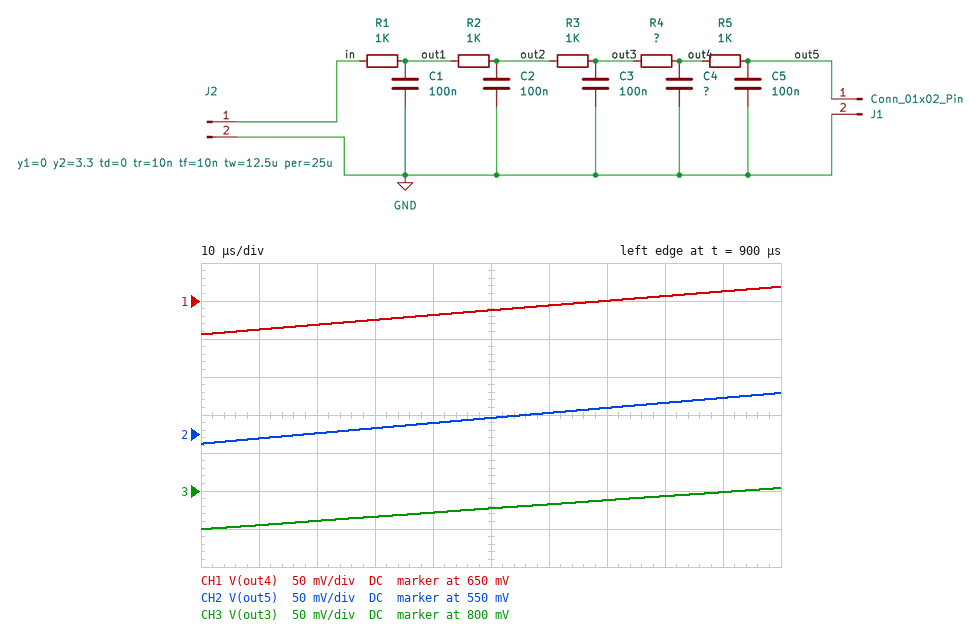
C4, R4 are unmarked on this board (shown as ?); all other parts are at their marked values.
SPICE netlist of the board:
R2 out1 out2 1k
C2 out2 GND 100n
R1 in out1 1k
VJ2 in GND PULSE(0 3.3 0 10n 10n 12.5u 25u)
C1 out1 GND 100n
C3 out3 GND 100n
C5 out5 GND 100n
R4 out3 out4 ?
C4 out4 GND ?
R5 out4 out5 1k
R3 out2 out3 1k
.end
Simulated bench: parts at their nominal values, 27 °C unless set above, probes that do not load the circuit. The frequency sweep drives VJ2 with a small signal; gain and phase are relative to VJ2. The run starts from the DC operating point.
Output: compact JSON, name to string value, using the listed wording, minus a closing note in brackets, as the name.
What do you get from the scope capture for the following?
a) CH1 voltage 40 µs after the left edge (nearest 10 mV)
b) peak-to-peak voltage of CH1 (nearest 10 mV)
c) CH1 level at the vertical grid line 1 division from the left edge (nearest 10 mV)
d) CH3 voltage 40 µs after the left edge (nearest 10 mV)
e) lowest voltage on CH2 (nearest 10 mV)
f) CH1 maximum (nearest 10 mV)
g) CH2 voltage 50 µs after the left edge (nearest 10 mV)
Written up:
{"CH1 voltage 40 µs after the left edge": "630 mV", "peak-to-peak voltage of CH1": "60 mV", "CH1 level at the vertical grid line 1 division from the left edge": "610 mV", "CH3 voltage 40 µs after the left edge": "770 mV", "lowest voltage on CH2": "540 mV", "CH1 maximum": "670 mV", "CH2 voltage 50 µs after the left edge": "570 mV"}
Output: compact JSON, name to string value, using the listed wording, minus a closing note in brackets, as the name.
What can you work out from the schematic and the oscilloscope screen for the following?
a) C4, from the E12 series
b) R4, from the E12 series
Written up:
{"C4, from the E12 series": "220 nF", "R4, from the E12 series": "680 Ω"}
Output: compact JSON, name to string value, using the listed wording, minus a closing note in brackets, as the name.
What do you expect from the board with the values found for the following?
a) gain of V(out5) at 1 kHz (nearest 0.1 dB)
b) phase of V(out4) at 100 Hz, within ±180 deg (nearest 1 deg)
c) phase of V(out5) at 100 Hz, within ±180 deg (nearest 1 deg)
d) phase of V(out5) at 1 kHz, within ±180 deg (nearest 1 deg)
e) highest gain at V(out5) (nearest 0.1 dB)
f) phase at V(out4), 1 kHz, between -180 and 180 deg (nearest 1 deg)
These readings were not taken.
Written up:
{"gain of V(out5) at 1 kHz": "-23.5 dB", "phase of V(out4) at 100 Hz, within ±180 deg": "-51 deg", "phase of V(out5) at 100 Hz, within ±180 deg": "-55 deg", "phase of V(out5) at 1 kHz, within ±180 deg": "-170 deg", "highest gain at V(out5)": "0 dB", "phase at V(out4), 1 kHz, between -180 and 180 deg": "-138 deg"}
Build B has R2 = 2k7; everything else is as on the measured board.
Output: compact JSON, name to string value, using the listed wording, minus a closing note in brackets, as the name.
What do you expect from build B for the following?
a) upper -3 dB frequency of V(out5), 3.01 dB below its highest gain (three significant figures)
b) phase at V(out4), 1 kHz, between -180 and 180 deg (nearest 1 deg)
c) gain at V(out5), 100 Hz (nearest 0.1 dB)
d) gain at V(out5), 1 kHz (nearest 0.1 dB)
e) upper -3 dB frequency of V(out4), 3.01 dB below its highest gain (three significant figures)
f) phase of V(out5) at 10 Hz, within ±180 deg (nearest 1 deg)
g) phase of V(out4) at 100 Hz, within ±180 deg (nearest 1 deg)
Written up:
{"upper -3 dB frequency of V(out5), 3.01 dB below its highest gain": "64.2 Hz", "phase at V(out4), 1 kHz, between -180 and 180 deg": "-149 deg", "gain at V(out5), 100 Hz": "-5.4 dB", "gain at V(out5), 1 kHz": "-27.7 dB", "upper -3 dB frequency of V(out4), 3.01 dB below its highest gain": "64.3 Hz", "phase of V(out5) at 10 Hz, within ±180 deg": "-10 deg", "phase of V(out4) at 100 Hz, within ±180 deg": "-64 deg"}
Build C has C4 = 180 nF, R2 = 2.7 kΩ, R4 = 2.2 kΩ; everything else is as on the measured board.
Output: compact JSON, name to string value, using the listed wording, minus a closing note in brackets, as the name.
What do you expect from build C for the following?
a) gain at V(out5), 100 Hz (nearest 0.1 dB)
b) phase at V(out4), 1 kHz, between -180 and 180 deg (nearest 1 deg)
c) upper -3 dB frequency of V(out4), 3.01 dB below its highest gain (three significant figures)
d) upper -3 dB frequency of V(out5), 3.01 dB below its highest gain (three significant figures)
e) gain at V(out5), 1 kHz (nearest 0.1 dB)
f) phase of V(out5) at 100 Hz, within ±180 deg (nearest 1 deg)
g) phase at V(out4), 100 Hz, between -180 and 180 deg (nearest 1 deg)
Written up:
{"gain at V(out5), 100 Hz": "-5.7 dB", "phase at V(out4), 1 kHz, between -180 and 180 deg": "-170 deg", "upper -3 dB frequency of V(out4), 3.01 dB below its highest gain": "61.6 Hz", "upper -3 dB frequency of V(out5), 3.01 dB below its highest gain": "61.5 Hz", "gain at V(out5), 1 kHz": "-30.9 dB", "phase of V(out5) at 100 Hz, within ±180 deg": "-73 deg", "phase at V(out4), 100 Hz, between -180 and 180 deg": "-69 deg"}
